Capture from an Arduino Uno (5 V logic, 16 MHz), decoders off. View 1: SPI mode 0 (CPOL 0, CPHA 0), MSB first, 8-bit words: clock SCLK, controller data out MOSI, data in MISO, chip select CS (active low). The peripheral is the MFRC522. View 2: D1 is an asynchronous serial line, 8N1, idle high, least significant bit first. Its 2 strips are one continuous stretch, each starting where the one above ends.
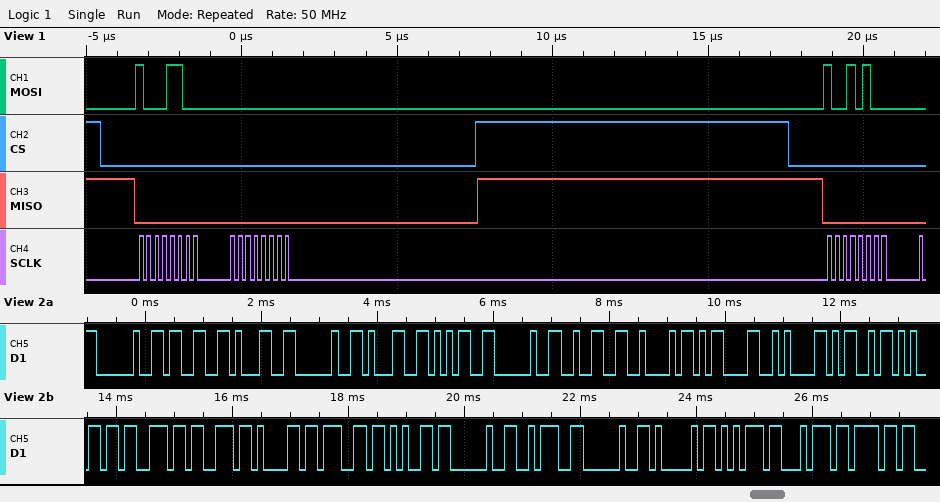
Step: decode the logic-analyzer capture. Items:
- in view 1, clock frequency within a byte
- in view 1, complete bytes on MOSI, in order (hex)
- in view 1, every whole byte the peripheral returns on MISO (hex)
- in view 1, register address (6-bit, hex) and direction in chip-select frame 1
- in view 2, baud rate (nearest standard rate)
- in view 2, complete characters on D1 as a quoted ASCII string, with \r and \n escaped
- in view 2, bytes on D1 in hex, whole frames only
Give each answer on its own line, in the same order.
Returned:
4 MHz
8C 00 94
00 00 00
0x06 read
9600 baud
" 31 15 2B\r\nMessage : Auto"
20 33 31 20 31 35 20 32 42 0D 0A 4D 65 73 73 61 67 65 20 3A 20 41 75 74 6F
